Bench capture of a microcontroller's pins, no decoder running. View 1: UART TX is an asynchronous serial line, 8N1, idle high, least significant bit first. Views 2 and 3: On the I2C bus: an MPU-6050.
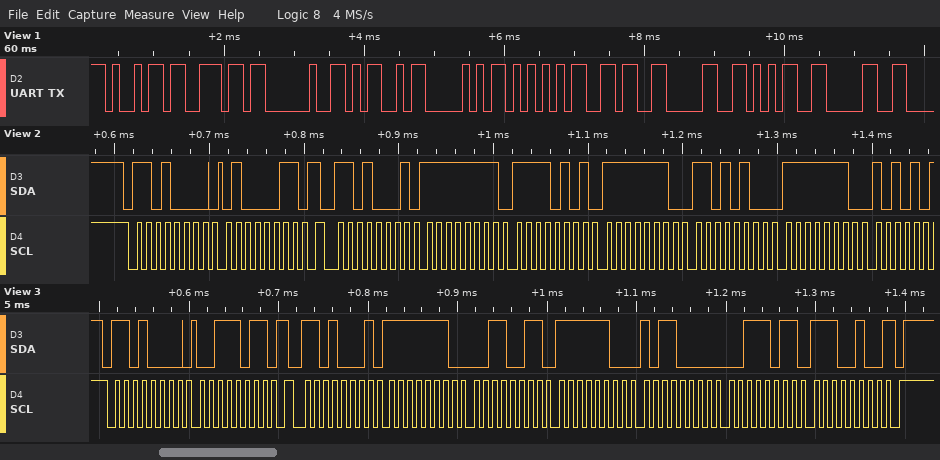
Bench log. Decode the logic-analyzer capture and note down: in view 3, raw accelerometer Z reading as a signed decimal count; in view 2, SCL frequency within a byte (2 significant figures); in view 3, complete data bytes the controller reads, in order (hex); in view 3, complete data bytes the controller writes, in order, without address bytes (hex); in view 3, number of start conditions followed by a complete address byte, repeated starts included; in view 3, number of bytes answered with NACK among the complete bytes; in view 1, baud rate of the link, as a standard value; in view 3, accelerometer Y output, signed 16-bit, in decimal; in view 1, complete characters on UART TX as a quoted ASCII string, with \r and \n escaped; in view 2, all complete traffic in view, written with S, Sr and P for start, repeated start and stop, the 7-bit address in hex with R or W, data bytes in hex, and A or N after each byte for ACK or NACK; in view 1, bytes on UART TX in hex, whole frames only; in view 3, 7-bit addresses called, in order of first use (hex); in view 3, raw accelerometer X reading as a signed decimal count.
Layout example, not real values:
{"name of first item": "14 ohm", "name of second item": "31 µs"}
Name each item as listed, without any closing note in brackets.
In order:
{"in view 3, raw accelerometer Z reading as a signed decimal count": "15332", "in view 2, SCL frequency within a byte": "100 kHz", "in view 3, complete data bytes the controller reads, in order": "FE 33 FC B0 3B E4", "in view 3, complete data bytes the controller writes, in order, without address bytes": "3B", "in view 3, number of start conditions followed by a complete address byte, repeated starts included": "2", "in view 3, number of bytes answered with NACK among the complete bytes": "1", "in view 1, baud rate of the link, as a standard value": "9600 baud", "in view 3, accelerometer Y output, signed 16-bit, in decimal": "-848", "in view 1, complete characters on UART TX as a quoted ASCII string, with \\r and \\n escaped": "\"in MPU6050\"", "in view 2, all complete traffic in view, written with S, Sr and P for start, repeated start and stop, the 7-bit address in hex with R or W, data bytes in hex, and A or N after each byte for ACK or NACK": "S 68W A 43 A Sr 68R A FF A F5 A FE A D4 A FE A", "in view 1, bytes on UART TX in hex, whole frames only": "0x69 0x6E 0x20 0x4D 0x50 0x55 0x36 0x30 0x35 0x30", "in view 3, 7-bit addresses called, in order of first use": "0x68", "in view 3, raw accelerometer X reading as a signed decimal count": "-461"}
